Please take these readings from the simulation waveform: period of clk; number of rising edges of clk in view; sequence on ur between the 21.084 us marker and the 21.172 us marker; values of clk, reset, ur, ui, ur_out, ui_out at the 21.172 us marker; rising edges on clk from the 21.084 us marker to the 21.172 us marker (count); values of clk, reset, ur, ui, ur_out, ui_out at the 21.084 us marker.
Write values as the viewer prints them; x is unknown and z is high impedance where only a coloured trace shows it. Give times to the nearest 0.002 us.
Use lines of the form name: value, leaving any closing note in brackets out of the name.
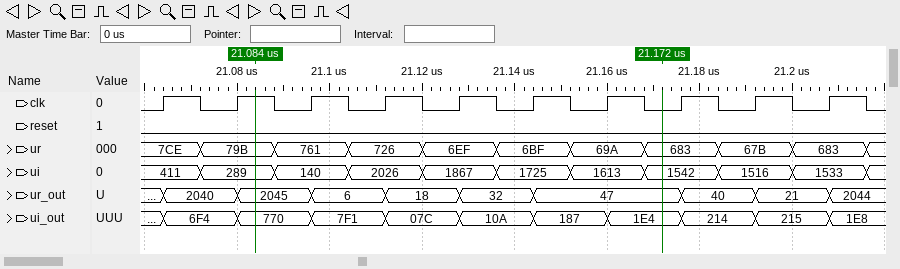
period of clk: 0.016 us
number of rising edges of clk in view: 10
sequence on ur between the 21.084 us marker and the 21.172 us marker: 79B, 761, 726, 6EF, 6BF, 69A, 683
values of clk, reset, ur, ui, ur_out, ui_out at the 21.172 us marker: clk=0, reset=0, ur=683, ui=1542, ur_out=47, ui_out=1E4
rising edges on clk from the 21.084 us marker to the 21.172 us marker: 5
values of clk, reset, ur, ui, ur_out, ui_out at the 21.084 us marker: clk=1, reset=0, ur=79B, ui=289, ur_out=2045, ui_out=770
